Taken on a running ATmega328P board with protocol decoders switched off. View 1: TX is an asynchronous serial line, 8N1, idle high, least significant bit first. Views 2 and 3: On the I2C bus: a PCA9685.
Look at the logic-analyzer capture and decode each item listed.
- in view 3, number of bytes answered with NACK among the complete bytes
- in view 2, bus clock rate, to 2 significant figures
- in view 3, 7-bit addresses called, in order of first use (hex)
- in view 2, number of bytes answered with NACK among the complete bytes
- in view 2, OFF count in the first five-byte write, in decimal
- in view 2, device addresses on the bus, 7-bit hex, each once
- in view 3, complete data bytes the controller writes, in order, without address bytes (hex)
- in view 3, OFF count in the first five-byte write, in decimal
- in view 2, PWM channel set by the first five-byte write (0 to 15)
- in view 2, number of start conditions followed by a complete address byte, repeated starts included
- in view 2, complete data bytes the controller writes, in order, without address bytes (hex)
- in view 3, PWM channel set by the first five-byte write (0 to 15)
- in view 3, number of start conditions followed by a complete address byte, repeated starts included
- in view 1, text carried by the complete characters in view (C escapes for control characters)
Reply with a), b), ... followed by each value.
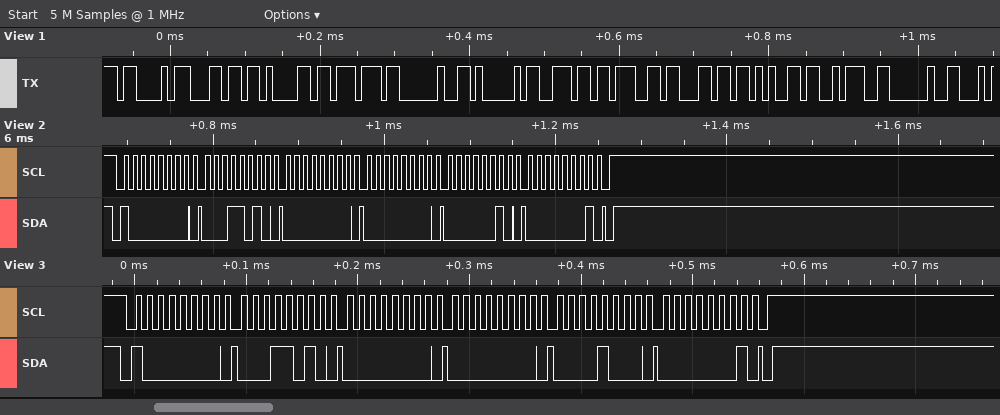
a) 0
b) 100 kHz
c) 0x40
d) 0
e) 258
f) 0x40
g) 1A 00 00 08 01
h) 264
i) 5
j) 1
k) 1A 00 00 02 01
l) 5
m) 1
n) "Claw Angle: "
